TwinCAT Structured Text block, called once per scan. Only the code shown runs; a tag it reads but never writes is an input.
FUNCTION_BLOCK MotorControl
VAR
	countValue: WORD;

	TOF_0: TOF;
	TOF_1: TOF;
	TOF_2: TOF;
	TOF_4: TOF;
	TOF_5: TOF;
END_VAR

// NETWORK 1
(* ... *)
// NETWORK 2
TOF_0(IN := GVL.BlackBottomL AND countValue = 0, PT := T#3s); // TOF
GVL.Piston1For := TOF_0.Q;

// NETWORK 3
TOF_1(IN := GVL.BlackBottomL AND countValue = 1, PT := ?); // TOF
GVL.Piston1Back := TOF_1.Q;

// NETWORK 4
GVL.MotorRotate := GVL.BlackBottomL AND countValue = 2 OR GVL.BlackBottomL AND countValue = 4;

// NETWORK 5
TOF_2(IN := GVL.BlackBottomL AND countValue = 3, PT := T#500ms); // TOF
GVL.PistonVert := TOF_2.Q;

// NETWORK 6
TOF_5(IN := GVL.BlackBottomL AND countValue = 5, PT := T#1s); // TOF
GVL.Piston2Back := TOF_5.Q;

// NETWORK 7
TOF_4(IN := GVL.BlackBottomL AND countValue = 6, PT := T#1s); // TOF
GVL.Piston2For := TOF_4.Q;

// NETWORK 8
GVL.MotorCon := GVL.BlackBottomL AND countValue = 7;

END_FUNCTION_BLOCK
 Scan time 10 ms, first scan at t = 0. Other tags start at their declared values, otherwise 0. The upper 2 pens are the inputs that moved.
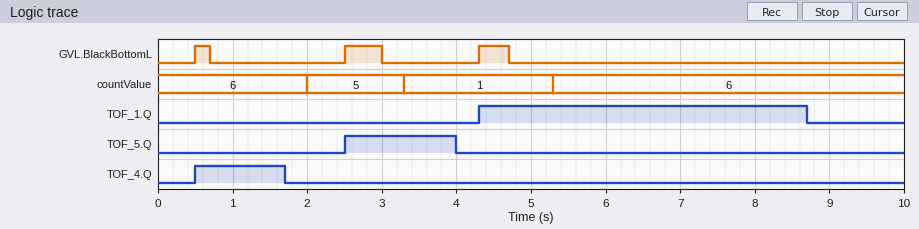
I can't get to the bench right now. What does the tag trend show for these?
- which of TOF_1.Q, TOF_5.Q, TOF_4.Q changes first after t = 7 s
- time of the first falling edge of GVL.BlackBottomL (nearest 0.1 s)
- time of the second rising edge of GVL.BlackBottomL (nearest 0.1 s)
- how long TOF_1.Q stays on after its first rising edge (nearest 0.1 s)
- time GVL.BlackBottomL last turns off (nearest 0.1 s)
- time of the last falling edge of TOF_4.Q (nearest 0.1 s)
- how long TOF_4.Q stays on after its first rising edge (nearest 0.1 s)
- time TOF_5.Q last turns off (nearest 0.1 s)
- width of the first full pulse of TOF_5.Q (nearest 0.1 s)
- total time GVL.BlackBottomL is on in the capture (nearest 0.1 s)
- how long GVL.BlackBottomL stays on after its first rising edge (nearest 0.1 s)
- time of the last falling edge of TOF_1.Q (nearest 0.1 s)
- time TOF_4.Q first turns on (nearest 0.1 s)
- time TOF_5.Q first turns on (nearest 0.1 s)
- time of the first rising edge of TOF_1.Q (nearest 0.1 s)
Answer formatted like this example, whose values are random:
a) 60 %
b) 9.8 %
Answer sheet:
a) TOF_1.Q
b) 0.7 s
c) 2.5 s
d) 4.4 s
e) 4.7 s
f) 1.7 s
g) 1.2 s
h) 4.0 s
i) 1.5 s
j) 1.1 s
k) 0.2 s
l) 8.7 s
m) 0.5 s
n) 2.5 s
o) 4.3 s
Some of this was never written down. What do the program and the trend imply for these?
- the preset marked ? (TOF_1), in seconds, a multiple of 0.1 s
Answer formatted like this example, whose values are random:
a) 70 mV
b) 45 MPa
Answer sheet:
a) 4.0 s
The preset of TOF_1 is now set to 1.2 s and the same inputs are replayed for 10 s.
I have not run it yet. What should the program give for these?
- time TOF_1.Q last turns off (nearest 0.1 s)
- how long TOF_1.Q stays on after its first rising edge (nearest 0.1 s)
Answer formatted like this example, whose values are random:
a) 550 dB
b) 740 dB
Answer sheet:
a) 5.9 s
b) 1.6 s
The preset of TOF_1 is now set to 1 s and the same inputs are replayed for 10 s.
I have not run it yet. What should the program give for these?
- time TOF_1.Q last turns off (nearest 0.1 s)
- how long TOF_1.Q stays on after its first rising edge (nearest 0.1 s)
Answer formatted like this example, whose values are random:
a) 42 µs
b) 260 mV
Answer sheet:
a) 5.7 s
b) 1.4 s
